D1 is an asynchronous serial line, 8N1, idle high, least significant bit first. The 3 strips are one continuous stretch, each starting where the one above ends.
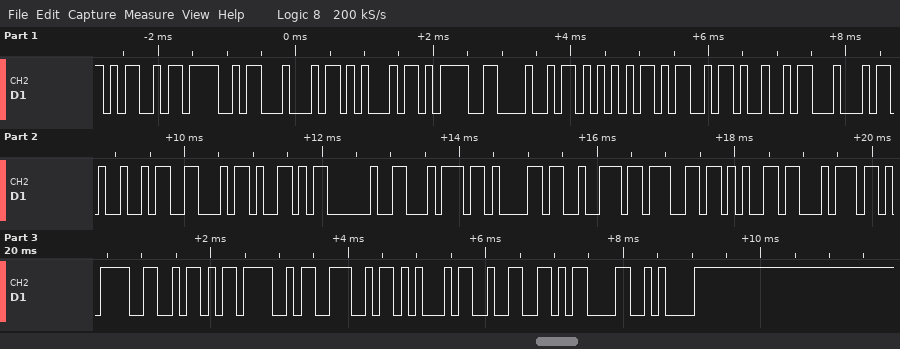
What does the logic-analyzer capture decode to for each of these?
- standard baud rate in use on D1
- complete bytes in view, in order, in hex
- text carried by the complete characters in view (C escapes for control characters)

9600 baud
4D 4F 44 45 3D 48 55 4D 49 44 49 46 59 20 74 61 72 67 65 74 3D 5A 4F 4E 45 32 0D 0A
"MODE=HUMIDIFY target=ZONE2\r\n"
